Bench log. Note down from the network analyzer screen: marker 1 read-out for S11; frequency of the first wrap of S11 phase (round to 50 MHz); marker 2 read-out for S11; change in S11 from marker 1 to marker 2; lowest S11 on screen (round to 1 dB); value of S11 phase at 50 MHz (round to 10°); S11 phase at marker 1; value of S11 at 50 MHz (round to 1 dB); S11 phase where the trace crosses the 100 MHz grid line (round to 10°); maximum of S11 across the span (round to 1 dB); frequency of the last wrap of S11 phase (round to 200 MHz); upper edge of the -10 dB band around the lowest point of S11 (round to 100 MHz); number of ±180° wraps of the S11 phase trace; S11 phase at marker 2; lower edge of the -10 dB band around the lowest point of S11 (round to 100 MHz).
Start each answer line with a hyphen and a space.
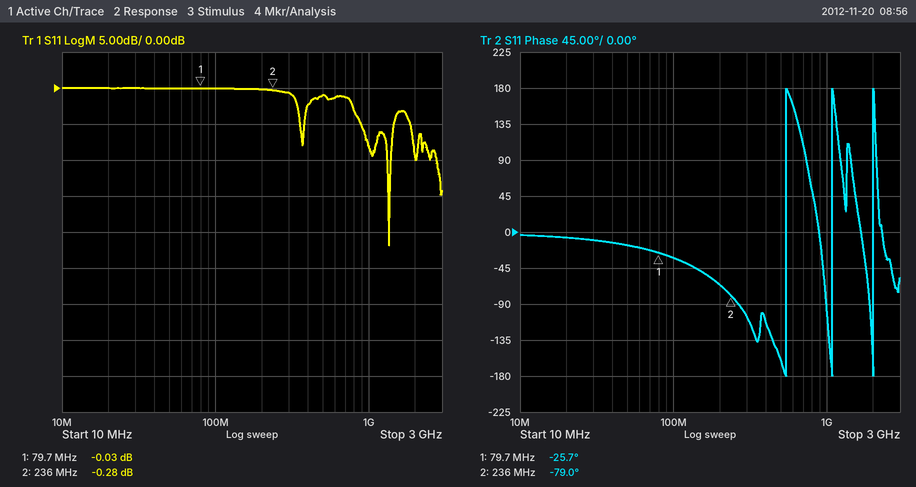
- -0.03 dB
- 550 MHz
- -0.28 dB
- -0.25 dB
- -22 dB
- -20°
- -25.7°
- 0 dB
- -30°
- 0 dB
- 2.0 GHz
- 1.4 GHz
- 3
- -79.0°
- 1.3 GHz
